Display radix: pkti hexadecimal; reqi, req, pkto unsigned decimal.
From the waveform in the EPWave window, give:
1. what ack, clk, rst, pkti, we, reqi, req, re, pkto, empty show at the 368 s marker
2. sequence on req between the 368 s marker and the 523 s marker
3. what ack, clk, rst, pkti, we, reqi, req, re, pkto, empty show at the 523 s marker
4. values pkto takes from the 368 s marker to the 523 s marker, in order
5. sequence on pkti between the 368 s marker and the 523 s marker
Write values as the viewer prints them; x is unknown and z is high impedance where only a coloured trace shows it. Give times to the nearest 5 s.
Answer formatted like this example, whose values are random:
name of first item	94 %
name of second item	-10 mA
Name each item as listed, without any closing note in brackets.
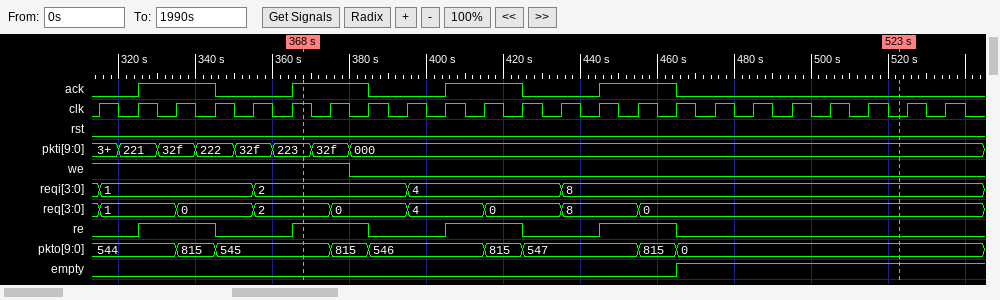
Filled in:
what ack, clk, rst, pkti, we, reqi, req, re, pkto, empty show at the 368 s marker	ack=1, clk=1, rst=0, pkti=223, we=1, reqi=2, req=2, re=1, pkto=545, empty=0
sequence on req between the 368 s marker and the 523 s marker	2, 0, 4, 0, 8, 0
what ack, clk, rst, pkti, we, reqi, req, re, pkto, empty show at the 523 s marker	ack=0, clk=0, rst=0, pkti=000, we=0, reqi=8, req=0, re=0, pkto=0, empty=1
values pkto takes from the 368 s marker to the 523 s marker, in order	545, 815, 546, 815, 547, 815, 0
sequence on pkti between the 368 s marker and the 523 s marker	223, 32f, 000
